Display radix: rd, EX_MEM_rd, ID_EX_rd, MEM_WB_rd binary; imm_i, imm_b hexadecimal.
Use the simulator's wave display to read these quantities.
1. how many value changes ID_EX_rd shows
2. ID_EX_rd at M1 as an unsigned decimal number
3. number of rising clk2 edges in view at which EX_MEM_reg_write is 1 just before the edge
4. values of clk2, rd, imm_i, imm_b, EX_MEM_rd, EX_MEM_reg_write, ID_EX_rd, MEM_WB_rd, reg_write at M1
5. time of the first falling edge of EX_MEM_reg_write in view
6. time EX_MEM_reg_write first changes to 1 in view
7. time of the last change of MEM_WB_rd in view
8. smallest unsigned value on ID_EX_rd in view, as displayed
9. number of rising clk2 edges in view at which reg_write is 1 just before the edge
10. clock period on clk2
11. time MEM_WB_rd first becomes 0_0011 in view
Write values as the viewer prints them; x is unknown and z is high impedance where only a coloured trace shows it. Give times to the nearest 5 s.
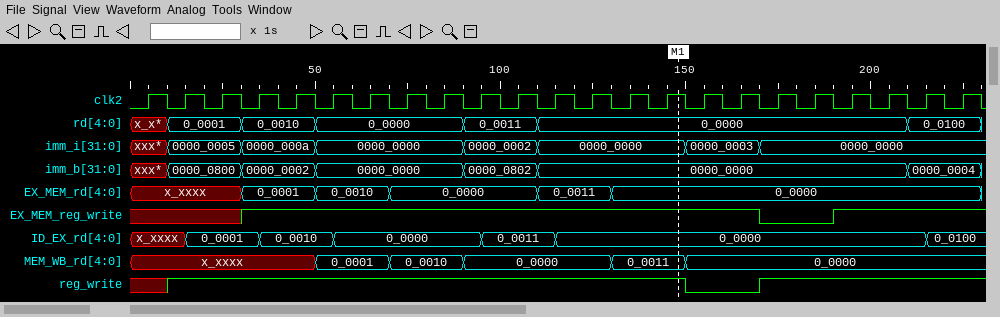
6
0
18
clk2=1, rd=0_0000, imm_i=0000_0000, imm_b=0000_0000, EX_MEM_rd=0_0000, EX_MEM_reg_write=1, ID_EX_rd=0_0000, MEM_WB_rd=0_0011, reg_write=1
170 s
30 s
150 s
0_0000
20
10 s
130 s
